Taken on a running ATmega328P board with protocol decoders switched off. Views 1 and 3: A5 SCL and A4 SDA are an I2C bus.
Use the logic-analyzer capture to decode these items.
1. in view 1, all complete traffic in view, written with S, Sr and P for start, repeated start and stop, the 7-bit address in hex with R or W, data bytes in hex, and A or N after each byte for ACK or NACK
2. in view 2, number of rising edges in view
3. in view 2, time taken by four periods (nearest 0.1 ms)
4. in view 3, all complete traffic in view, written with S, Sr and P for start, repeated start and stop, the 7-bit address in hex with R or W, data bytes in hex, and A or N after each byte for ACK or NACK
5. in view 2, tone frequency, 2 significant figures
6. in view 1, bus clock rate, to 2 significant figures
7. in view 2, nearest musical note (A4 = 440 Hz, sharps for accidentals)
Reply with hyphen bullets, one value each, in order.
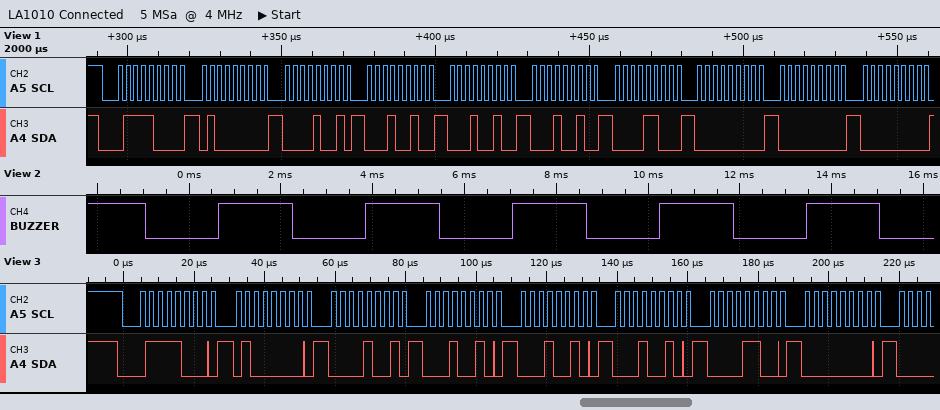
- S 3CW A 40 A 09 A 12 A 12 A 12 A 0C A 00 A 00 A 00 A
- 5
- 12.8 ms
- S 3CW A 40 A 09 A 12 A 12 A 12 A 0C A 00 A
- 310 Hz
- 400 kHz
- D#4
